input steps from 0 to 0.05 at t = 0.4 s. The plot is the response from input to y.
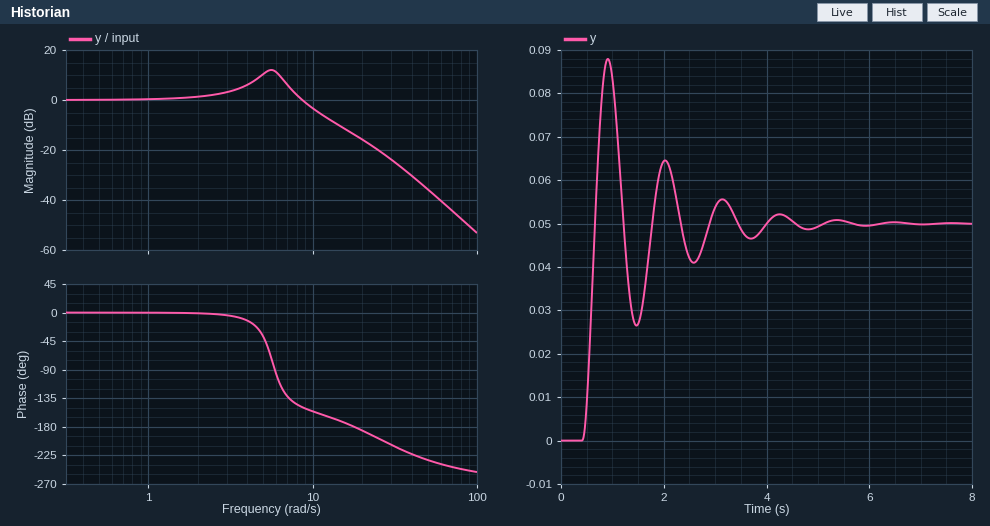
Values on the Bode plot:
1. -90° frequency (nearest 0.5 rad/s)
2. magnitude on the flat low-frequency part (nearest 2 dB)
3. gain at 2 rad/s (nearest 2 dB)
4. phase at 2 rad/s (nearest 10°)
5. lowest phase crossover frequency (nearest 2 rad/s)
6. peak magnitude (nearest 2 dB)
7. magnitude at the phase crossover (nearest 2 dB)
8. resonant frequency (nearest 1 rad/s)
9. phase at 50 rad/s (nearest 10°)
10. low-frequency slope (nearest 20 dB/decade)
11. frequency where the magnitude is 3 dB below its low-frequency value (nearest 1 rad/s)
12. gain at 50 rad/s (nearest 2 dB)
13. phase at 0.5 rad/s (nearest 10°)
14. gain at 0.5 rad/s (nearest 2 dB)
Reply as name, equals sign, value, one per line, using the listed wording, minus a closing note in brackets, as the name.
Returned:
-90° frequency = 6.0 rad/s
magnitude on the flat low-frequency part = 0 dB
gain at 2 rad/s = 2 dB
phase at 2 rad/s = 0°
lowest phase crossover frequency = 18 rad/s
peak magnitude = 12 dB
magnitude at the phase crossover = -14 dB
resonant frequency = 6 rad/s
phase at 50 rad/s = -230°
low-frequency slope = 0 dB/decade
frequency where the magnitude is 3 dB below its low-frequency value = 10 rad/s
gain at 50 rad/s = -36 dB
phase at 0.5 rad/s = 0°
gain at 0.5 rad/s = 0 dB
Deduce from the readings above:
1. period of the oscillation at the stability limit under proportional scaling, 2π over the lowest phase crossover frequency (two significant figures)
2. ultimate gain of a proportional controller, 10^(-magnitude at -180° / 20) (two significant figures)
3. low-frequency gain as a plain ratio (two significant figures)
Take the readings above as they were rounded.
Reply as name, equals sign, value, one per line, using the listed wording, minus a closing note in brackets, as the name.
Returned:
period of the oscillation at the stability limit under proportional scaling, 2π over the lowest phase crossover frequency = 0.35 s
ultimate gain of a proportional controller, 10^(-magnitude at -180° / 20) = 5.0
low-frequency gain as a plain ratio = 1.0
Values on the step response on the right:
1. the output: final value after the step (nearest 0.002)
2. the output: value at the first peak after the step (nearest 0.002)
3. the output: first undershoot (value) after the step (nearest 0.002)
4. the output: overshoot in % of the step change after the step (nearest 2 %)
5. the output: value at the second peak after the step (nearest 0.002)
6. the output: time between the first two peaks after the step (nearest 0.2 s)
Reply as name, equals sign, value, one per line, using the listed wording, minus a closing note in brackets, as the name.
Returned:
the output: final value after the step = 0.050
the output: value at the first peak after the step = 0.088
the output: first undershoot (value) after the step = 0.026
the output: overshoot in % of the step change after the step = 76 %
the output: value at the second peak after the step = 0.064
the output: time between the first two peaks after the step = 1.2 s
